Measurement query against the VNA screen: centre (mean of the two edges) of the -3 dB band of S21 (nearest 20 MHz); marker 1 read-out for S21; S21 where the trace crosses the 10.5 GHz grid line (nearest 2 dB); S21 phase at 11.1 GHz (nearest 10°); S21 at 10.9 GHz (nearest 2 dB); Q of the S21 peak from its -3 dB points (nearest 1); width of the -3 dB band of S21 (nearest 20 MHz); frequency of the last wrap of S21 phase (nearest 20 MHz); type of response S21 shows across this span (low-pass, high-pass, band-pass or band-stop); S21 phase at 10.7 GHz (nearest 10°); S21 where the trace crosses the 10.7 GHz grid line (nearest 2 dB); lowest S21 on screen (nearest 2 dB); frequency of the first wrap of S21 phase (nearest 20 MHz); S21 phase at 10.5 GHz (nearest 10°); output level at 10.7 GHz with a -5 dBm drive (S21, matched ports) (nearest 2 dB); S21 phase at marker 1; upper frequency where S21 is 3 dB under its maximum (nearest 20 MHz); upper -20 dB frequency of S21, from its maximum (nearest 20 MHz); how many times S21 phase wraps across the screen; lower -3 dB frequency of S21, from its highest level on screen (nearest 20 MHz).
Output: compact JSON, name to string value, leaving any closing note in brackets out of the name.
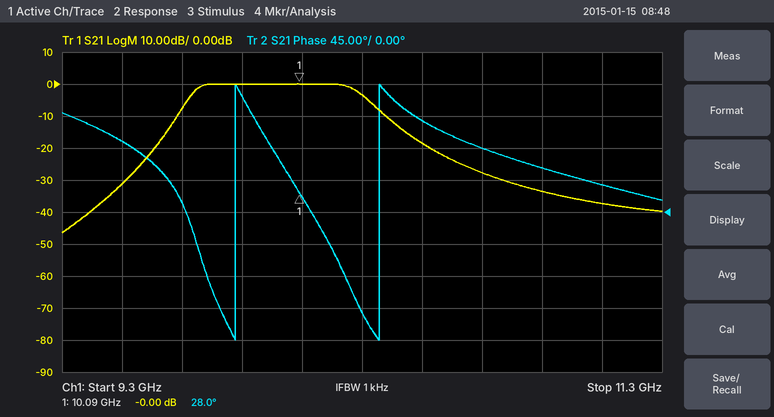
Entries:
{"centre (mean of the two edges) of the -3 dB band of S21": "10.02 GHz", "marker 1 read-out for S21": "-0.00 dB", "S21 where the trace crosses the 10.5 GHz grid line": "-18 dB", "S21 phase at 11.1 GHz": "40°", "S21 at 10.9 GHz": "-34 dB", "Q of the S21 peak from its -3 dB points": "18", "width of the -3 dB band of S21": "560 MHz", "frequency of the last wrap of S21 phase": "10.36 GHz", "type of response S21 shows across this span": "band-pass", "S21 phase at 10.7 GHz": "90°", "S21 where the trace crosses the 10.7 GHz grid line": "-28 dB", "lowest S21 on screen": "-46 dB", "frequency of the first wrap of S21 phase": "9.88 GHz", "S21 phase at 10.5 GHz": "130°", "output level at 10.7 GHz with a -5 dBm drive (S21, matched ports)": "-32 dBm", "S21 phase at marker 1": "28.0°", "upper frequency where S21 is 3 dB under its maximum": "10.30 GHz", "upper -20 dB frequency of S21, from its maximum": "10.52 GHz", "how many times S21 phase wraps across the screen": "2", "lower -3 dB frequency of S21, from its highest level on screen": "9.74 GHz"}
